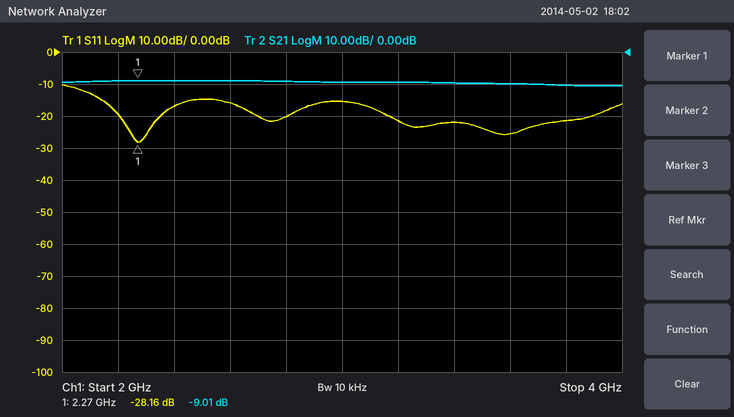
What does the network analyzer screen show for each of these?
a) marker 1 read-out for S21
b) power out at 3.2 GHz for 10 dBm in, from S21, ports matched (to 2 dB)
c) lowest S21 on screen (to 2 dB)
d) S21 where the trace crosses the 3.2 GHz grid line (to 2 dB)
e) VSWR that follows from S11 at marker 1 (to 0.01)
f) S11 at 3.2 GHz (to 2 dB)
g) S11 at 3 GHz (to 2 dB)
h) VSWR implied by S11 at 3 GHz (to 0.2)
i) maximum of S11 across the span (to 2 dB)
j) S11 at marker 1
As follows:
-9.01 dB
0 dBm
-10 dB
-10 dB
1.08
-22 dB
-16 dB
1.4
-10 dB
-28.16 dB
